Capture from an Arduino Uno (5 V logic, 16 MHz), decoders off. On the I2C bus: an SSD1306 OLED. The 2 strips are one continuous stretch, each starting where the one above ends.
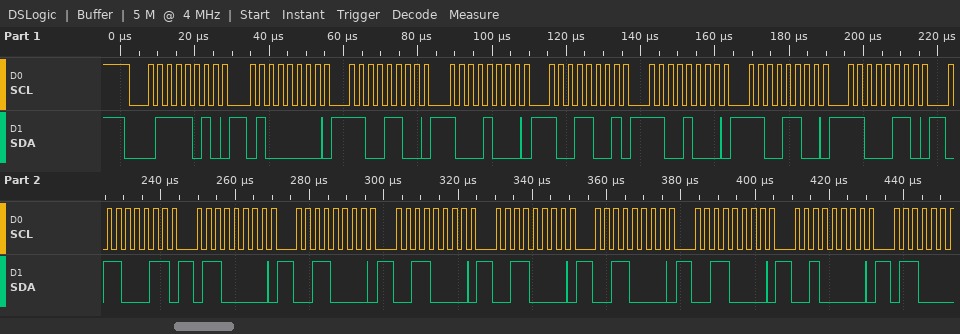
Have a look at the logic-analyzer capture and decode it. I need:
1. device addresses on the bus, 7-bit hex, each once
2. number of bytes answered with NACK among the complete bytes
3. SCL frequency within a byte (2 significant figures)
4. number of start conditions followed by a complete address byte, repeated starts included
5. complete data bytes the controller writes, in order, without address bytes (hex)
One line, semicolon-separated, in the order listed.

0x3D; 0; 400 kHz; 1; 40 CC 88 99 C8 CC C6 63 60 30 30 30 30 30 20
